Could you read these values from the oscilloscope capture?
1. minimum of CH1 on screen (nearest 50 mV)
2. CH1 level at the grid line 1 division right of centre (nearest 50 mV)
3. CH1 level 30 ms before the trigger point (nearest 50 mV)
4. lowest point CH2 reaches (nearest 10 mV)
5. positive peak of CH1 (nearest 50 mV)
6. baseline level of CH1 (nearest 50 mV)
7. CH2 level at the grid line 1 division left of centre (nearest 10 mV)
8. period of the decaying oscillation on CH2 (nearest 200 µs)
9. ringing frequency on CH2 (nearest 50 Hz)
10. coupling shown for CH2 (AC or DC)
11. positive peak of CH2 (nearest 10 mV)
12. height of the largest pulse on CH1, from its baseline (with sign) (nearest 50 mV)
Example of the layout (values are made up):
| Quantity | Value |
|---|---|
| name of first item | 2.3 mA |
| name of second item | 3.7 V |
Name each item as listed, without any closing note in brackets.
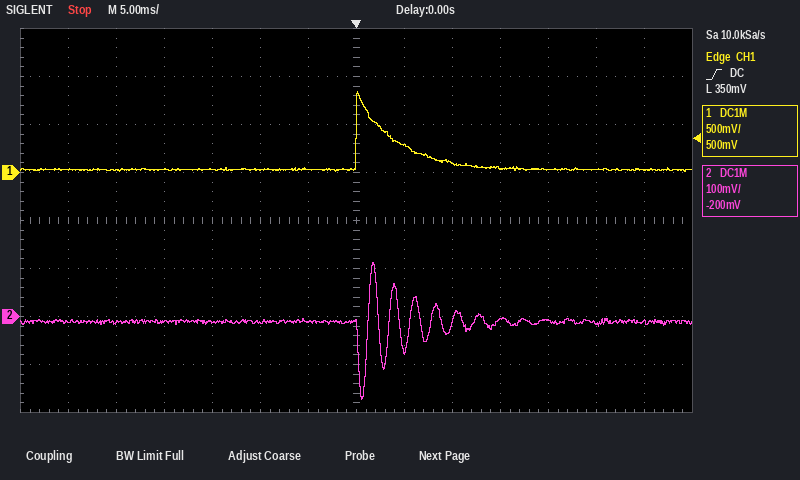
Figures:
| Quantity | Value |
|---|---|
| minimum of CH1 on screen | 0 mV |
| CH1 level at the grid line 1 division right of centre | 300 mV |
| CH1 level 30 ms before the trigger point | 50 mV |
| lowest point CH2 reaches | -170 mV |
| positive peak of CH1 | 850 mV |
| baseline level of CH1 | 50 mV |
| CH2 level at the grid line 1 division left of centre | -10 mV |
| period of the decaying oscillation on CH2 | 2.2 ms |
| ringing frequency on CH2 | 450 Hz |
| coupling shown for CH2 | DC |
| positive peak of CH2 | 110 mV |
| height of the largest pulse on CH1, from its baseline (with sign) | +800 mV |
